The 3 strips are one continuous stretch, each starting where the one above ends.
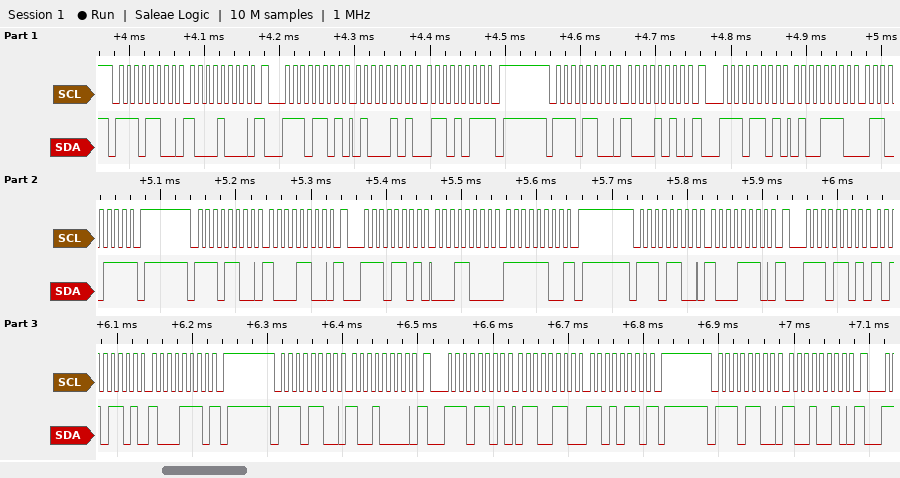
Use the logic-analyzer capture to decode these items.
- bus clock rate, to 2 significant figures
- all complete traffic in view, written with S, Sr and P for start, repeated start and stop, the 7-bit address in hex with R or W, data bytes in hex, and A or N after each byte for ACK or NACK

100 kHz
S 76W A 88 A Sr 76R A 45 A 6B N P S 76W A 8A A Sr 76R A 4E A 67 N P S 76W A 8C A Sr 76R A 18 A FC N P S 76W A 8E A Sr 76R A AD A 8E N P S 76W A 90 A Sr 76R A 66 A D6 N P S 76W A 92 A
